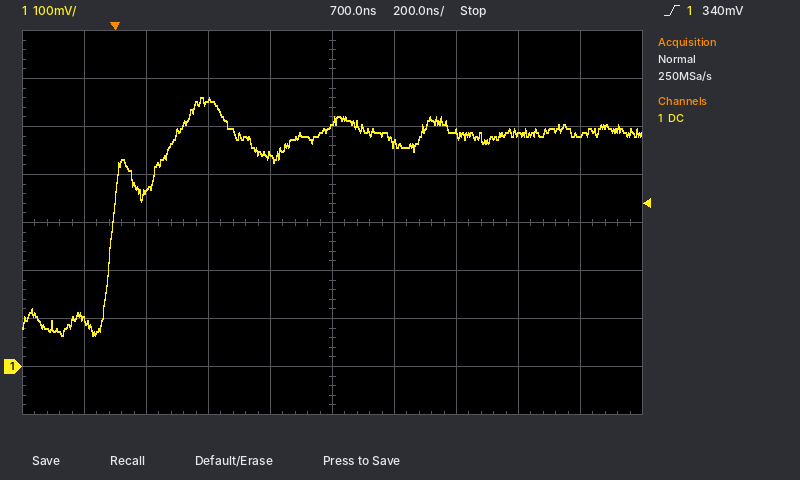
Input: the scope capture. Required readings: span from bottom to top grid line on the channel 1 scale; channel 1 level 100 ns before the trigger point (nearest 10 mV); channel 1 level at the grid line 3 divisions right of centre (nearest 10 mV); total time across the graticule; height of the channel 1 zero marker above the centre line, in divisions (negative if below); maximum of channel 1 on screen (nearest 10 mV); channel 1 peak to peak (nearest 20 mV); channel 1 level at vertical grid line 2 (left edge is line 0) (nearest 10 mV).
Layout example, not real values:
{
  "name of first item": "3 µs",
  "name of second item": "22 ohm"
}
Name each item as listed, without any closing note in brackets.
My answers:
{
  "span from bottom to top grid line on the channel 1 scale": "800 mV",
  "channel 1 level 100 ns before the trigger point": "100 mV",
  "channel 1 level at the grid line 3 divisions right of centre": "490 mV",
  "total time across the graticule": "2 µs",
  "height of the channel 1 zero marker above the centre line, in divisions": "-3.0 div",
  "maximum of channel 1 on screen": "560 mV",
  "channel 1 peak to peak": "500 mV",
  "channel 1 level at vertical grid line 2 (left edge is line 0)": "370 mV"
}
